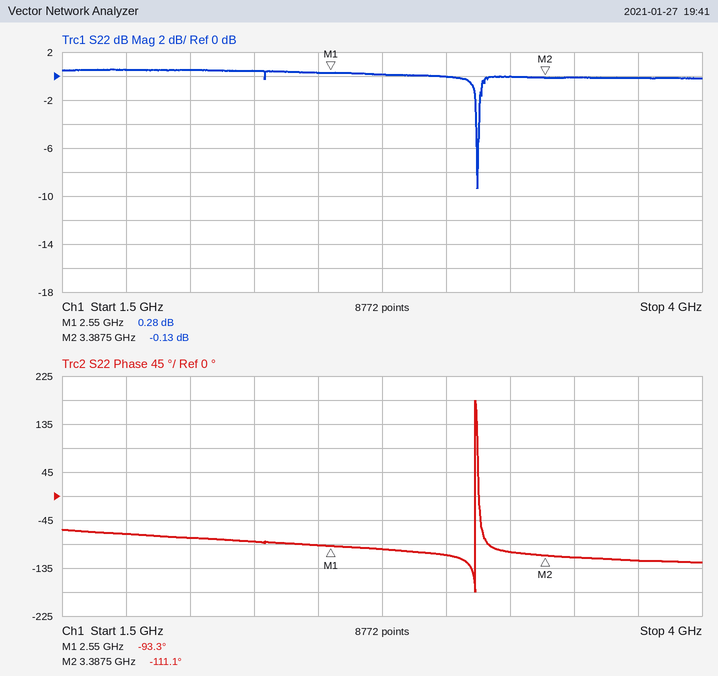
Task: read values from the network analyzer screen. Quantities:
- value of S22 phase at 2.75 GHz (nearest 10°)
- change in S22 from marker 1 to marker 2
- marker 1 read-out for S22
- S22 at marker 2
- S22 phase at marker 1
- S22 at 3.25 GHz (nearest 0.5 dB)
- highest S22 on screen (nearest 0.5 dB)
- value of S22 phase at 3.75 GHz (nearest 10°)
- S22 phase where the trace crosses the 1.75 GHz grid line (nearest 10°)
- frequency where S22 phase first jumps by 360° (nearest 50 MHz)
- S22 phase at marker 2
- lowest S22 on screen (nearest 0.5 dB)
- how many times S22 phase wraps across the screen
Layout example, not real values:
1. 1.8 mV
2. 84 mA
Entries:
1. -100°
2. -0.41 dB
3. 0.28 dB
4. -0.13 dB
5. -93.3°
6. 0.0 dB
7. 0.5 dB
8. -120°
9. -70°
10. 3.10 GHz
11. -111.1°
12. -9.5 dB
13. 1
